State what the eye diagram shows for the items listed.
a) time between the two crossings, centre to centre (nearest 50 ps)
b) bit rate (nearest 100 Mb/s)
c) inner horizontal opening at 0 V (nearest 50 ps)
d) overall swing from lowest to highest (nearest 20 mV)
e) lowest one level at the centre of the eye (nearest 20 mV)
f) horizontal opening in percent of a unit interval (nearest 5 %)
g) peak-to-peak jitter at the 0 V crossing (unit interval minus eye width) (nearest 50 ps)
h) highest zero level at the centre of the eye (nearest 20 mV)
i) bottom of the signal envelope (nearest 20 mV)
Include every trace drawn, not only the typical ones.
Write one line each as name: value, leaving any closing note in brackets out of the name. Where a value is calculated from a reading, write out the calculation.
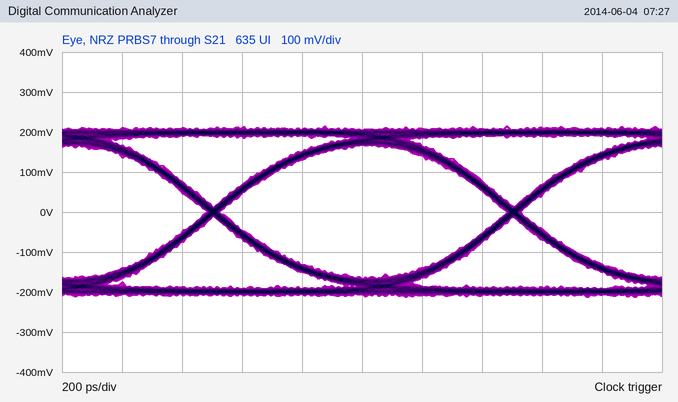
time between the two crossings, centre to centre: 1.00 ns
bit rate: 1.0 Gb/s
inner horizontal opening at 0 V: 950 ps
overall swing from lowest to highest: 420 mV
lowest one level at the centre of the eye: 160 mV
horizontal opening in percent of a unit interval: 950 ps / 1.00 ns ≈ 95 %
peak-to-peak jitter at the 0 V crossing (unit interval minus eye width): 50 ps
highest zero level at the centre of the eye: -160 mV
bottom of the signal envelope: -220 mV
